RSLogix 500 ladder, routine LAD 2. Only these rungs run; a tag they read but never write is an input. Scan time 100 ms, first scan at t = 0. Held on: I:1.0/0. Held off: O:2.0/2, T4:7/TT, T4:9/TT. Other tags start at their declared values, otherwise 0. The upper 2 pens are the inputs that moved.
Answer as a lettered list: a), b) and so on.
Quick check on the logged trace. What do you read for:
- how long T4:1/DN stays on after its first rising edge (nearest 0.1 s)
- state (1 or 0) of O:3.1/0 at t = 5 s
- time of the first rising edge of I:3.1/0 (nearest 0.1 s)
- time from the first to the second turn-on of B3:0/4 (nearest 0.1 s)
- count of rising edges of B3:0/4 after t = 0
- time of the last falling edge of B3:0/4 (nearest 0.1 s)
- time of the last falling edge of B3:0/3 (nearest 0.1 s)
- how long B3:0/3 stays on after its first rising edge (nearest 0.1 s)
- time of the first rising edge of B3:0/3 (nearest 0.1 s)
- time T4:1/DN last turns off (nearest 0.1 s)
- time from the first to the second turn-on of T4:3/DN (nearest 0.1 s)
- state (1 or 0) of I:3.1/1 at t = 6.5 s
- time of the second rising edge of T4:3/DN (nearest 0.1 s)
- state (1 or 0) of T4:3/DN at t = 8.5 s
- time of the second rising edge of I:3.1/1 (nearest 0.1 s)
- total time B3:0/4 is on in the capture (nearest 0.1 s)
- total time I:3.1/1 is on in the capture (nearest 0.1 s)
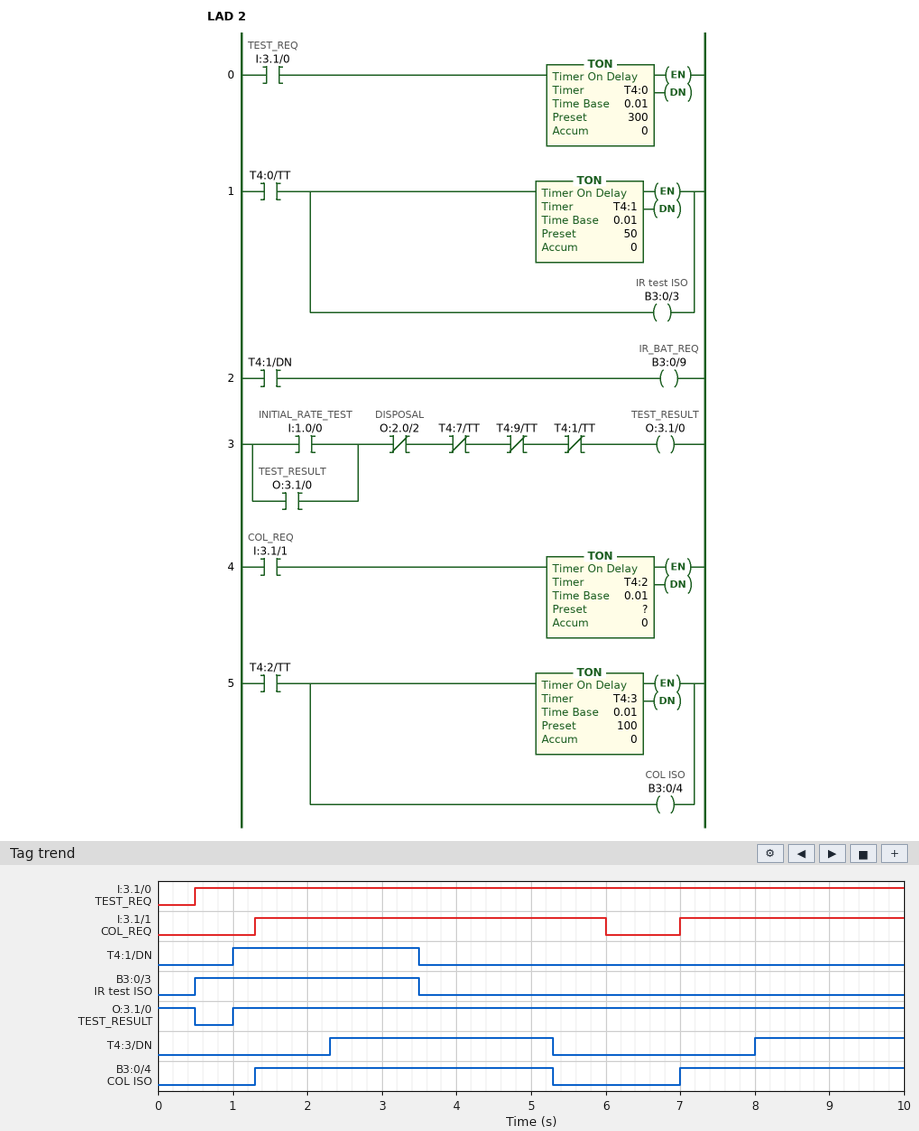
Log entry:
a) 2.5 s
b) 1
c) 0.5 s
d) 5.7 s
e) 2
f) 5.3 s
g) 3.5 s
h) 3.0 s
i) 0.5 s
j) 3.5 s
k) 5.7 s
l) 0
m) 8.0 s
n) 1
o) 7.0 s
p) 7.0 s
q) 7.7 s
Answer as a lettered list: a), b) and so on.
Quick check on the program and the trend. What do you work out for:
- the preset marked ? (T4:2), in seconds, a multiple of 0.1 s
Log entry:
a) 4.0 s
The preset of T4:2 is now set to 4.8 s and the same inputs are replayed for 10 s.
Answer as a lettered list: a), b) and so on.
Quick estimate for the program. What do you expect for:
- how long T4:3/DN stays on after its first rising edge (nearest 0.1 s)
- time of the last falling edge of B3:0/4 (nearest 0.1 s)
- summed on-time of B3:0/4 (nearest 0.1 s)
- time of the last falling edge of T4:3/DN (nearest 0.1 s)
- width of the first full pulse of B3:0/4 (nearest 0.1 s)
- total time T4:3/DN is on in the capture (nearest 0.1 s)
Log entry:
a) 3.7 s
b) 6.0 s
c) 7.7 s
d) 6.0 s
e) 4.7 s
f) 5.7 s
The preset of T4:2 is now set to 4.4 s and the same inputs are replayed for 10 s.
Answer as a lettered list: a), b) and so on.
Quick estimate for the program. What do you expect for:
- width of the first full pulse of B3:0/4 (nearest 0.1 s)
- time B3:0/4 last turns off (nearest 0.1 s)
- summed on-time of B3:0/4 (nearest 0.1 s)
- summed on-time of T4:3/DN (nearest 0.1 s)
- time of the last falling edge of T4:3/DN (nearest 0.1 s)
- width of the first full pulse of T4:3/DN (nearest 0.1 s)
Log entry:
a) 4.4 s
b) 5.7 s
c) 7.4 s
d) 5.4 s
e) 5.7 s
f) 3.4 s
